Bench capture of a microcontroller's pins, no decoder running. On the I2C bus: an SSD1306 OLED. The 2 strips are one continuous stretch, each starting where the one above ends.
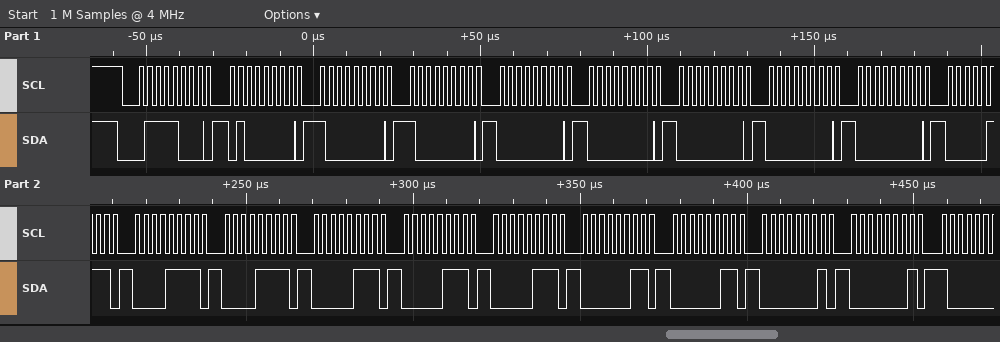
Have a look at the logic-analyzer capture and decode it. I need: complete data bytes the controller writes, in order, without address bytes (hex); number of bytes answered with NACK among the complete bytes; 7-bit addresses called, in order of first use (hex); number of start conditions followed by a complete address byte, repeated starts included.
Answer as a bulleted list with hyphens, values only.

- 40 80 80 00 00 00 00 00 07 0F 0F 07 07 07 03 03 01 01
- 0
- 0x3C
- 1
